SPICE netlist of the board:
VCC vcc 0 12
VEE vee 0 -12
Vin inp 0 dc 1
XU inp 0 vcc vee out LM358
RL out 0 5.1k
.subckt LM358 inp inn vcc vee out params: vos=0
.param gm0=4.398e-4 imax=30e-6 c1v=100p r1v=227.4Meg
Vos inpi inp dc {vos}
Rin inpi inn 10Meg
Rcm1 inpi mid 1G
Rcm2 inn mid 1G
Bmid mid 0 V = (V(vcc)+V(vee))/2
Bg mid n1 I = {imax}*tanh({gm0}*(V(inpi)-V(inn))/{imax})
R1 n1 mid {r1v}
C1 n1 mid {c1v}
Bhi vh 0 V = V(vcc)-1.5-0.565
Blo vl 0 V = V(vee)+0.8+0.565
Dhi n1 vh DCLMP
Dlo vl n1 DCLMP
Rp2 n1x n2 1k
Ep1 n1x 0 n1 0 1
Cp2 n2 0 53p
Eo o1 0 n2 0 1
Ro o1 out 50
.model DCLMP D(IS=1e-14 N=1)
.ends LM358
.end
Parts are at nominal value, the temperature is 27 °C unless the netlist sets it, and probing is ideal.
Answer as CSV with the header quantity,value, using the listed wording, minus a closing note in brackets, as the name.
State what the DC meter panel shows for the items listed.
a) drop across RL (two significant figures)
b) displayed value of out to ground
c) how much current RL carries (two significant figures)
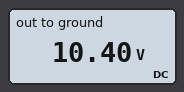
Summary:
quantity,value
drop across RL,10 V
displayed value of out to ground,10.40 V
how much current RL carries,2.0 mA
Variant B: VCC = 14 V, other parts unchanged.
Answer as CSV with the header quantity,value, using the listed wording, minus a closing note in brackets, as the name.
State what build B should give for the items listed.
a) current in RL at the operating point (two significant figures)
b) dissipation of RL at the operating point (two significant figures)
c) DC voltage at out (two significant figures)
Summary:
quantity,value
current in RL at the operating point,2.4 mA
dissipation of RL at the operating point,30 mW
DC voltage at out,12 V
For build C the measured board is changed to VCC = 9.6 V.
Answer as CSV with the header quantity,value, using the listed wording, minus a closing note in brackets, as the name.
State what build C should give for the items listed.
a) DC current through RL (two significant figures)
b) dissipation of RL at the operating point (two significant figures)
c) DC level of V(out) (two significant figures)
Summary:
quantity,value
DC current through RL,1.6 mA
dissipation of RL at the operating point,13 mW
DC level of V(out),8.0 V
